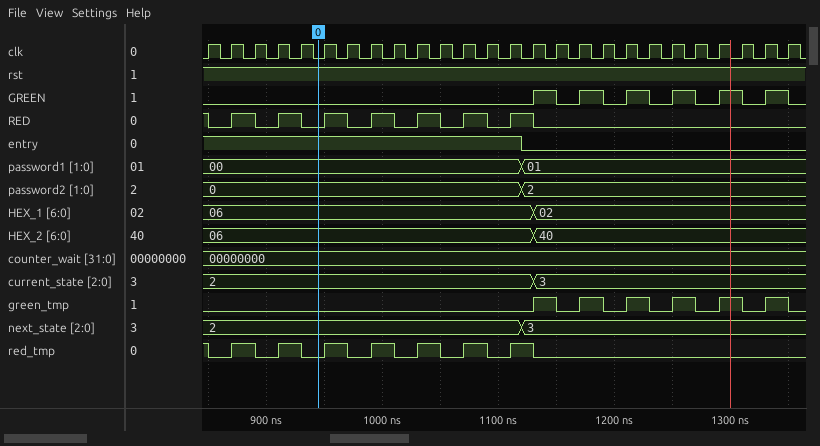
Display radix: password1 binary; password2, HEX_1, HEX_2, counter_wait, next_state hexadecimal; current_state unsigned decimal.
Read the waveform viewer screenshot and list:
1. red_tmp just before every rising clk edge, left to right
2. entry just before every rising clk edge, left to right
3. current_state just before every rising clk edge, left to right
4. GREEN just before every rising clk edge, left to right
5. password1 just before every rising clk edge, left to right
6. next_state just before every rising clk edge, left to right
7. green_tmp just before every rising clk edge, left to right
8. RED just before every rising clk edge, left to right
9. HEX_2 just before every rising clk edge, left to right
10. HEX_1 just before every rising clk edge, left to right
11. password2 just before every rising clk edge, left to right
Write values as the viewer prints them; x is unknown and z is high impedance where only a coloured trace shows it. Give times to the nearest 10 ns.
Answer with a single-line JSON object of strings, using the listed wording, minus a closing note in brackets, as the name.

{"red_tmp just before every rising clk edge, left to right": "1 0 1 0 1 0 1 0 1 0 1 0 1 0 1 0 0 0 0 0 0 0 0 0 0 0", "entry just before every rising clk edge, left to right": "1 1 1 1 1 1 1 1 1 1 1 1 1 1 0 0 0 0 0 0 0 0 0 0 0 0", "current_state just before every rising clk edge, left to right": "2, 2, 2, 2, 2, 2, 2, 2, 2, 2, 2, 2, 2, 2, 2, 3, 3, 3, 3, 3, 3, 3, 3, 3, 3, 3", "GREEN just before every rising clk edge, left to right": "0 0 0 0 0 0 0 0 0 0 0 0 0 0 0 1 0 1 0 1 0 1 0 1 0 1", "password1 just before every rising clk edge, left to right": "00, 00, 00, 00, 00, 00, 00, 00, 00, 00, 00, 00, 00, 00, 01, 01, 01, 01, 01, 01, 01, 01, 01, 01, 01, 01", "next_state just before every rising clk edge, left to right": "2, 2, 2, 2, 2, 2, 2, 2, 2, 2, 2, 2, 2, 2, 3, 3, 3, 3, 3, 3, 3, 3, 3, 3, 3, 3", "green_tmp just before every rising clk edge, left to right": "0 0 0 0 0 0 0 0 0 0 0 0 0 0 0 1 0 1 0 1 0 1 0 1 0 1", "RED just before every rising clk edge, left to right": "1 0 1 0 1 0 1 0 1 0 1 0 1 0 1 0 0 0 0 0 0 0 0 0 0 0", "HEX_2 just before every rising clk edge, left to right": "06, 06, 06, 06, 06, 06, 06, 06, 06, 06, 06, 06, 06, 06, 06, 40, 40, 40, 40, 40, 40, 40, 40, 40, 40, 40", "HEX_1 just before every rising clk edge, left to right": "06, 06, 06, 06, 06, 06, 06, 06, 06, 06, 06, 06, 06, 06, 06, 02, 02, 02, 02, 02, 02, 02, 02, 02, 02, 02", "password2 just before every rising clk edge, left to right": "0, 0, 0, 0, 0, 0, 0, 0, 0, 0, 0, 0, 0, 0, 2, 2, 2, 2, 2, 2, 2, 2, 2, 2, 2, 2"}
